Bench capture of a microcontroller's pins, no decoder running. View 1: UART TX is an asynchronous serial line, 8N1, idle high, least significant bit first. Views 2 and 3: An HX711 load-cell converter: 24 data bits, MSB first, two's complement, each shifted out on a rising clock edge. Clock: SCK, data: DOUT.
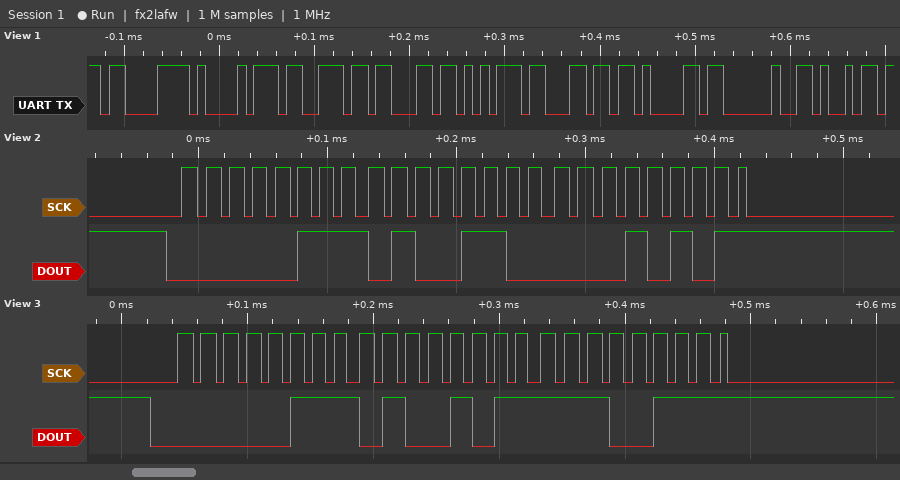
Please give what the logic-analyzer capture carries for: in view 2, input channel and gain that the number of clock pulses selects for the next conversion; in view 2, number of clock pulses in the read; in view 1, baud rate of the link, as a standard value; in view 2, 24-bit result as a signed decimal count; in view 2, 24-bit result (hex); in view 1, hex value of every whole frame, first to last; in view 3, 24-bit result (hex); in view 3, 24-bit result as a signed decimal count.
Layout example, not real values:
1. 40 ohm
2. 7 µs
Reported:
1. channel A, gain 128
2. 25
3. 115200 baud
4. 478229
5. 0x074C15
6. 0xC3 0xA1 0x73 0x63 0x75 0x6C 0x61 0x20 0x69
7. 0x074BE7
8. 478183
